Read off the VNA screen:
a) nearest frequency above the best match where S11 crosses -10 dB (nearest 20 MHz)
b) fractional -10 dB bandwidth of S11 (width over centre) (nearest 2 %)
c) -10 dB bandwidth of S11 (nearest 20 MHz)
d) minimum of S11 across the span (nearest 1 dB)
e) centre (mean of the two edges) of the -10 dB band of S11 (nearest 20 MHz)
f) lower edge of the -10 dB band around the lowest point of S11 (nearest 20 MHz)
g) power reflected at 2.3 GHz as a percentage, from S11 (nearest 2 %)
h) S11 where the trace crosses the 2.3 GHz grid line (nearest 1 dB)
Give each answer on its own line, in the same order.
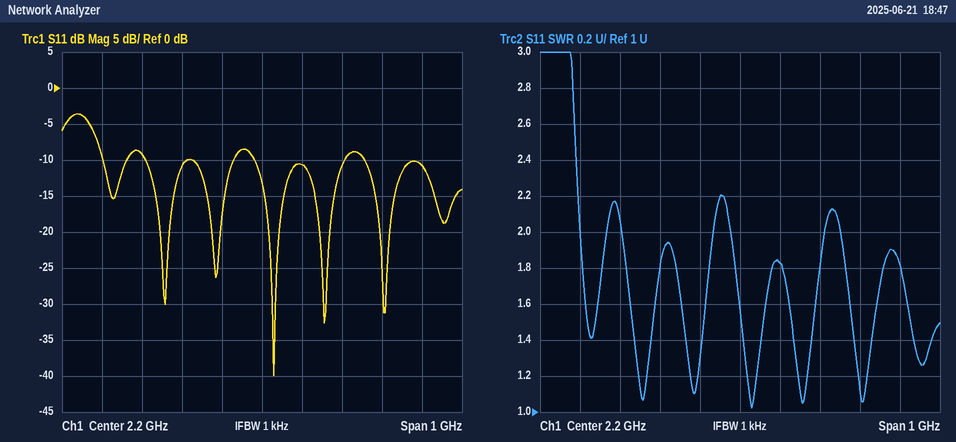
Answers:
2.40 GHz
10 %
220 MHz
-40 dB
2.30 GHz
2.18 GHz
8 %
-11 dB
